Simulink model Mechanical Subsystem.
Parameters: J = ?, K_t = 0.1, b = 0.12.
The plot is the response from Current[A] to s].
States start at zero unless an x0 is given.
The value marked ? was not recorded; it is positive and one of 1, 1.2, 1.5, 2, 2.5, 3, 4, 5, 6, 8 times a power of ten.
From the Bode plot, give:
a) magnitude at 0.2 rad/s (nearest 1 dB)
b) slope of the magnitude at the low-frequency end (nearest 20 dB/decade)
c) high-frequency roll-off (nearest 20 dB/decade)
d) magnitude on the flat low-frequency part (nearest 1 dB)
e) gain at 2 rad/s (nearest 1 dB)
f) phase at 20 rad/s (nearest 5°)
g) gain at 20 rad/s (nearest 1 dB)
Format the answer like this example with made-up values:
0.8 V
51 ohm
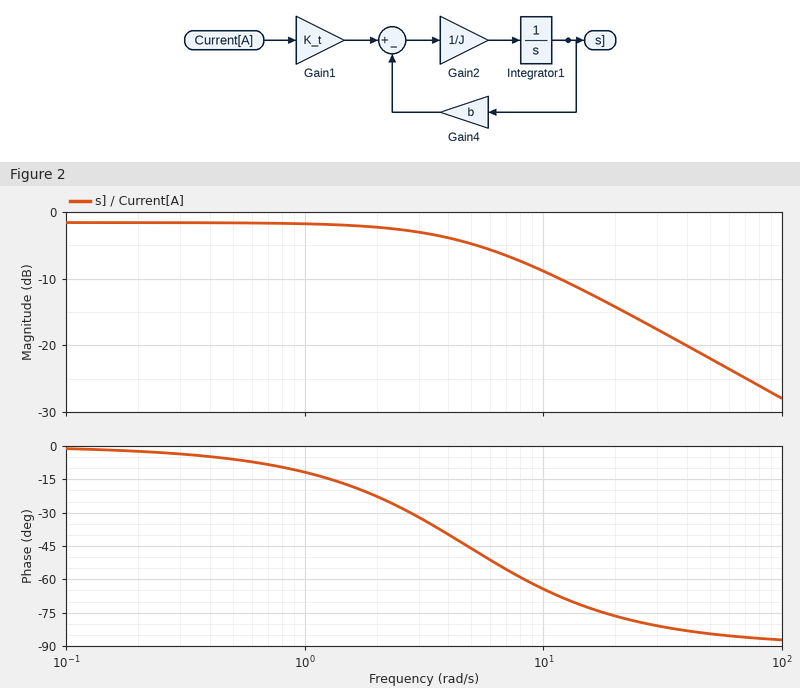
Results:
-2 dB
0 dB/decade
-20 dB/decade
-2 dB
-2 dB
-75°
-14 dB
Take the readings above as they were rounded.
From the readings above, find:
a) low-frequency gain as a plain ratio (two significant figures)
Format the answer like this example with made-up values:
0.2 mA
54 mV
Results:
0.79
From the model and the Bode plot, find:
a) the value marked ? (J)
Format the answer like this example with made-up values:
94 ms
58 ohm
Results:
0.025
